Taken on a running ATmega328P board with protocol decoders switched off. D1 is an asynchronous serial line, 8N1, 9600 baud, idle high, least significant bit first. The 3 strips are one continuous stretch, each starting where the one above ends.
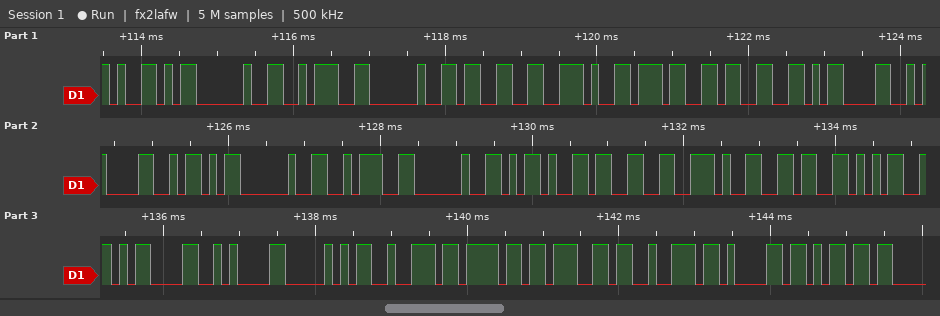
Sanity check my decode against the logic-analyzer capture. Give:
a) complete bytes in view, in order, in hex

59 20 3A 20 33 2E 37 33 0D 0A 5A 20 3A 20 2D 33 2E 36 35 0D 0A 50 72 6F 67 72 61 6D
